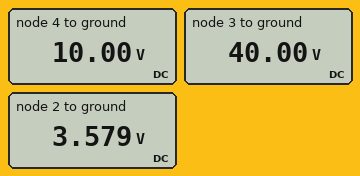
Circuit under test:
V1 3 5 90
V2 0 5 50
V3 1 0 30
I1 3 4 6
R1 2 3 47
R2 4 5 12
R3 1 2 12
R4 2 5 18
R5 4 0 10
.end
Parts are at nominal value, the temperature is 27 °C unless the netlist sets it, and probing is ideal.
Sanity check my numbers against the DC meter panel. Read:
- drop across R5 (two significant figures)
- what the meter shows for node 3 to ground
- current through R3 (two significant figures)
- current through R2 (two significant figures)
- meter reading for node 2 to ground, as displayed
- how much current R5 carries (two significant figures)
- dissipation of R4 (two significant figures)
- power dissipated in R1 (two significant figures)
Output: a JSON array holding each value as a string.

["10 V", "40.00 V", "2.2 A", "5.0 A", "3.579 V", "1.0 A", "160 W", "28 W"]
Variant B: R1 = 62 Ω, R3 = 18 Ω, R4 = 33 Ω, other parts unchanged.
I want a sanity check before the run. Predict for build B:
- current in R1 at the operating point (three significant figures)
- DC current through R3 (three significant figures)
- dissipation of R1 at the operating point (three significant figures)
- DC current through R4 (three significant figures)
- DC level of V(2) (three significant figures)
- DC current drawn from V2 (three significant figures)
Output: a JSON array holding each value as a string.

["519 mA", "1.23 A", "16.7 W", "1.75 A", "7.81 V", "233 mA"]
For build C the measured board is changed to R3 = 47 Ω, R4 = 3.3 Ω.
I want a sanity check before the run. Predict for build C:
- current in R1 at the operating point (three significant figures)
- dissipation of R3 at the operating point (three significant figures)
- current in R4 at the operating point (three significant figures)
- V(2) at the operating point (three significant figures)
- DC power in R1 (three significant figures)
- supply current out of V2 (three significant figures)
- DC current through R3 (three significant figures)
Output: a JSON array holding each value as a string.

["1.69 A", "103 W", "3.17 A", "-39.5 V", "135 W", "479 mA", "1.48 A"]
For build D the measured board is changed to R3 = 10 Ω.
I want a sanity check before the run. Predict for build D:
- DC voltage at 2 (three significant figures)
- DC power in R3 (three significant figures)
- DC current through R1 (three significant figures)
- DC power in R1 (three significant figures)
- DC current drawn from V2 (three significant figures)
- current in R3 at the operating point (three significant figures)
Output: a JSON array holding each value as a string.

["6.07 V", "57.3 W", "722 mA", "24.5 W", "1.39 A", "2.39 A"]
